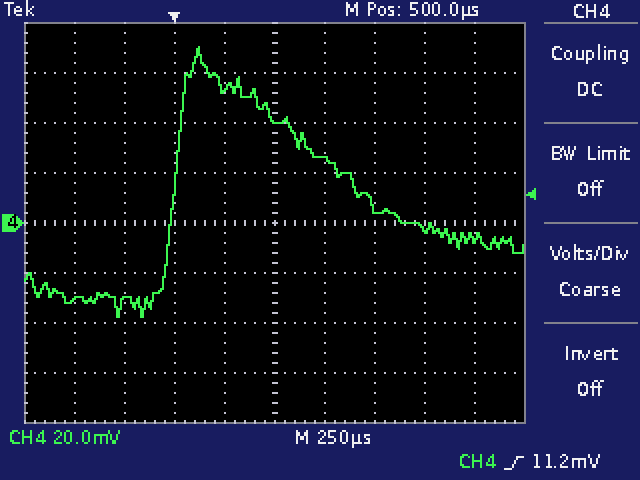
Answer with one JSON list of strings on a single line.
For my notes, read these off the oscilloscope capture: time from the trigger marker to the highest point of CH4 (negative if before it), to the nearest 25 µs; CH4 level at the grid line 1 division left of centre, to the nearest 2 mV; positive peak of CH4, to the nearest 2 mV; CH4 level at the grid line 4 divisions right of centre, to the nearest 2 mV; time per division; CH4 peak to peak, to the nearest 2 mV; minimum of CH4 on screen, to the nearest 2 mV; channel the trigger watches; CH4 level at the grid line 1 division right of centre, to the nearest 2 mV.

["+125 µs", "54 mV", "70 mV", "-6 mV", "250 µs", "108 mV", "-38 mV", "CH4", "26 mV"]
